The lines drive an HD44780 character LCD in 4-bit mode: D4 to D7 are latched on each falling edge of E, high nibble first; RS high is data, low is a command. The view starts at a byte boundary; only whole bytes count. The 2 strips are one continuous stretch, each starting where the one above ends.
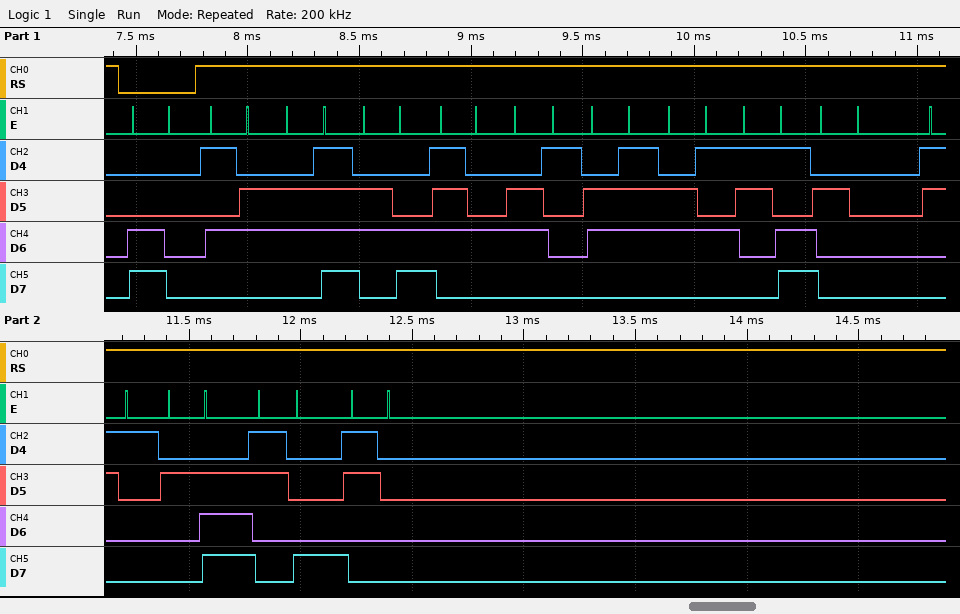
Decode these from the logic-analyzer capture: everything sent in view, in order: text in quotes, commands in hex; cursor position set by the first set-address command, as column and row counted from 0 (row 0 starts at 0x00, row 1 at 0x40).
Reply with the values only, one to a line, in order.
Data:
0xC0 "Voltage= 1.80"
column 0, row 1
